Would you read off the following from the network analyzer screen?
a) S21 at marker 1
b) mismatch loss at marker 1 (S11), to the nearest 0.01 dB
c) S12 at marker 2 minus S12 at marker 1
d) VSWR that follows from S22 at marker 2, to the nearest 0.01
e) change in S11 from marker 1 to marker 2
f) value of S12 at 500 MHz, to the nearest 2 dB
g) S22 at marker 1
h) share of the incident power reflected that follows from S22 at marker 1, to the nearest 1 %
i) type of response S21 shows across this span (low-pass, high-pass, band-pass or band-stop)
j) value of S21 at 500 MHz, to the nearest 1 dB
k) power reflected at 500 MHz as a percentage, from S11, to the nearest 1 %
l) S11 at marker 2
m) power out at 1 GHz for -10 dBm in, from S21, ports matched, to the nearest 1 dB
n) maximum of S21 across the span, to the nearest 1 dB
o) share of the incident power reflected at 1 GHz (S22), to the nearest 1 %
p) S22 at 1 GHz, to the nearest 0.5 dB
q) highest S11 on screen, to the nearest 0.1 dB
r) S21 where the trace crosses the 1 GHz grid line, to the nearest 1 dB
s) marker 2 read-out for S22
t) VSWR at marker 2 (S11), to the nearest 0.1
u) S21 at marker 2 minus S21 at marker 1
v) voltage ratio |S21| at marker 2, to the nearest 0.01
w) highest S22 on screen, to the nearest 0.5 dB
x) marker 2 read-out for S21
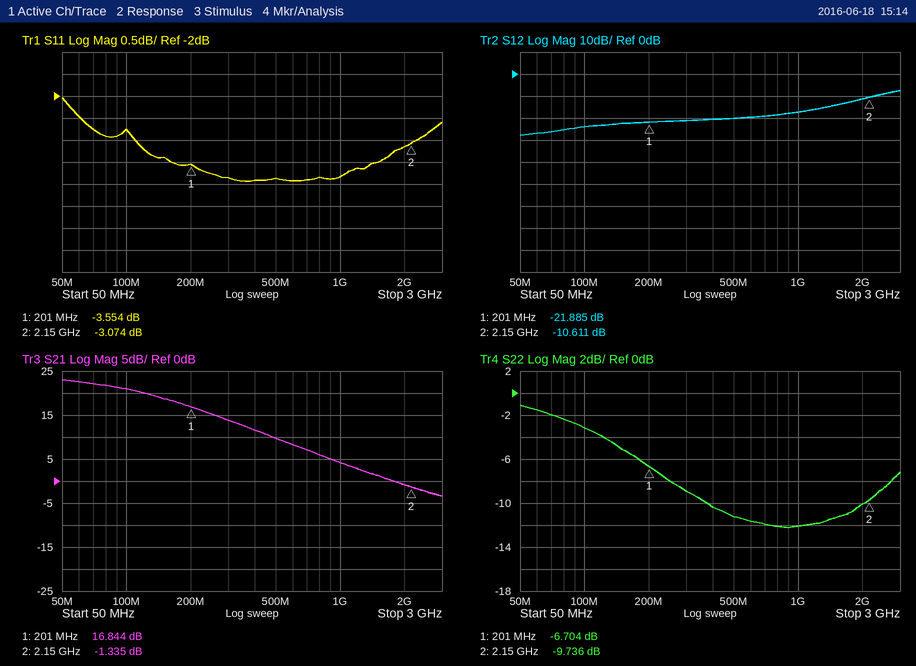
16.844 dB
2.53 dB
11.274 dB
1.97
0.480 dB
-20 dB
-6.704 dB
21 %
low-pass
10 dB
41 %
-3.074 dB
-6 dBm
23 dB
6 %
-12.0 dB
-2.0 dB
4 dB
-9.736 dB
5.7
-18.179 dB
0.86
-1.0 dB
-1.335 dB
